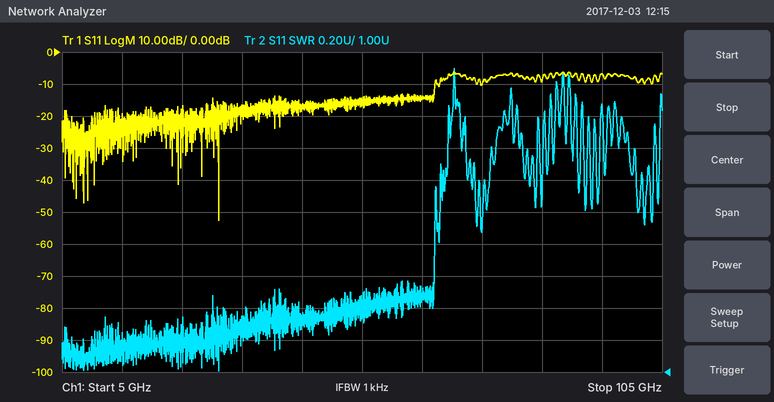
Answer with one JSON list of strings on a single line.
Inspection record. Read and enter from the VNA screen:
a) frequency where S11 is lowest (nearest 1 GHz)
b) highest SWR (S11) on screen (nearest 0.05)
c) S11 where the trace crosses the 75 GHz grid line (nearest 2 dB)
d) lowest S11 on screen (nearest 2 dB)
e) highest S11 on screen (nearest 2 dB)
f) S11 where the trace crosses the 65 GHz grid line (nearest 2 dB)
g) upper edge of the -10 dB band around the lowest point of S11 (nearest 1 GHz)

["31 GHz", "2.90", "-10 dB", "-52 dB", "-6 dB", "-14 dB", "67 GHz"]
